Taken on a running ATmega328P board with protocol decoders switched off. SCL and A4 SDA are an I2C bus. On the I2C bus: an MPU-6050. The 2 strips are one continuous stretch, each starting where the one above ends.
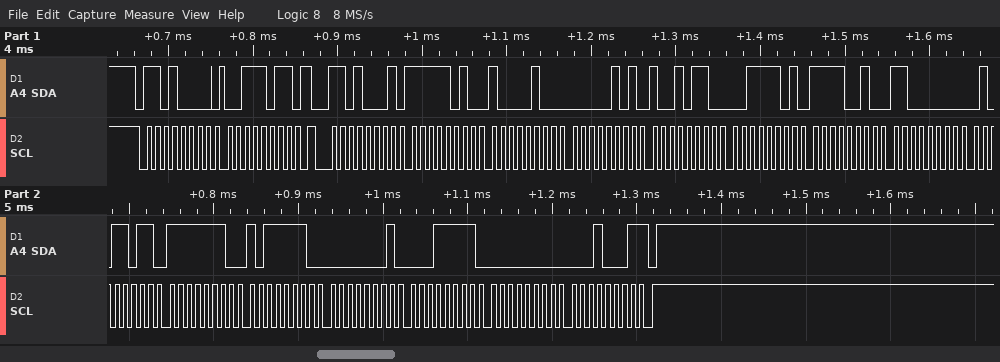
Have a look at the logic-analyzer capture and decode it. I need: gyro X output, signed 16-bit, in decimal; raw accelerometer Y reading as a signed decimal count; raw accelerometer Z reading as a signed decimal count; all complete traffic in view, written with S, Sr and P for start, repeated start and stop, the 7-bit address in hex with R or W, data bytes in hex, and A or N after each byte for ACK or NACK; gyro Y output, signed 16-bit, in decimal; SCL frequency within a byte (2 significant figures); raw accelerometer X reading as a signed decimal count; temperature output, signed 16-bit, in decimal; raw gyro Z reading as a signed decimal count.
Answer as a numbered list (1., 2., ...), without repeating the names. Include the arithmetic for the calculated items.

1. 0xFEBE = -322
2. 0x0596 = 1430
3. 0x3DF2 = 15858
4. S 68W A 3B A Sr 68R A FA A 84 A 05 A 96 A 3D A F2 A C0 A 5B A FE A BE A 01 A 1F A 00 A 11 N P
5. 0x011F = 287
6. 100 kHz
7. 0xFA84 = -1404
8. 0xC05B = -16293
9. 0x0011 = 17
